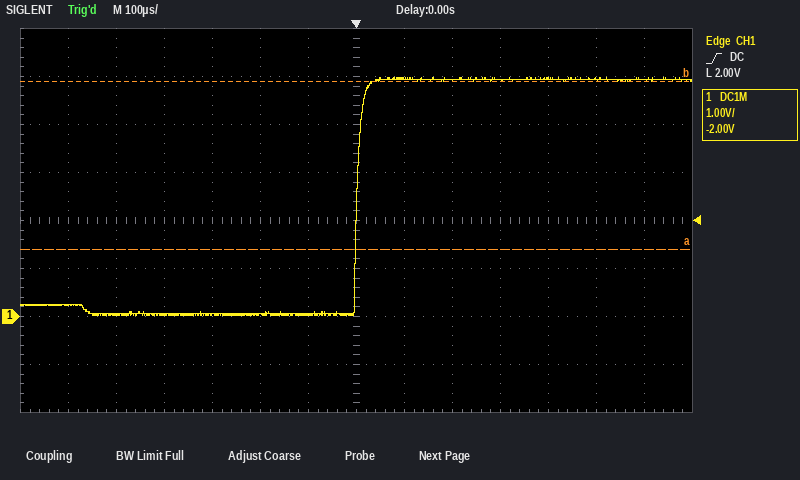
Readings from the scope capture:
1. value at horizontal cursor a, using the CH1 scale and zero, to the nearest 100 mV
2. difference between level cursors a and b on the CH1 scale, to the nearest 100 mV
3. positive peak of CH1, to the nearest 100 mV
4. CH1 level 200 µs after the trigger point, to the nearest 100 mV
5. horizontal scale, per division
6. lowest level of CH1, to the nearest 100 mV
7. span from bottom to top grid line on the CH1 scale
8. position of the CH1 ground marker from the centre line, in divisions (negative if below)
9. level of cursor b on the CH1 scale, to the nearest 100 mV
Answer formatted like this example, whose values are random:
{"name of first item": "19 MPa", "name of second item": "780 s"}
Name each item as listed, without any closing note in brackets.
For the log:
{"value at horizontal cursor a, using the CH1 scale and zero, to the nearest 100 mV": "1.4 V", "difference between level cursors a and b on the CH1 scale, to the nearest 100 mV": "3.5 V", "positive peak of CH1, to the nearest 100 mV": "5.0 V", "CH1 level 200 µs after the trigger point, to the nearest 100 mV": "4.9 V", "horizontal scale, per division": "100 µs", "lowest level of CH1, to the nearest 100 mV": "0.0 V", "span from bottom to top grid line on the CH1 scale": "8 V", "position of the CH1 ground marker from the centre line, in divisions": "-2.0 div", "level of cursor b on the CH1 scale, to the nearest 100 mV": "4.9 V"}
